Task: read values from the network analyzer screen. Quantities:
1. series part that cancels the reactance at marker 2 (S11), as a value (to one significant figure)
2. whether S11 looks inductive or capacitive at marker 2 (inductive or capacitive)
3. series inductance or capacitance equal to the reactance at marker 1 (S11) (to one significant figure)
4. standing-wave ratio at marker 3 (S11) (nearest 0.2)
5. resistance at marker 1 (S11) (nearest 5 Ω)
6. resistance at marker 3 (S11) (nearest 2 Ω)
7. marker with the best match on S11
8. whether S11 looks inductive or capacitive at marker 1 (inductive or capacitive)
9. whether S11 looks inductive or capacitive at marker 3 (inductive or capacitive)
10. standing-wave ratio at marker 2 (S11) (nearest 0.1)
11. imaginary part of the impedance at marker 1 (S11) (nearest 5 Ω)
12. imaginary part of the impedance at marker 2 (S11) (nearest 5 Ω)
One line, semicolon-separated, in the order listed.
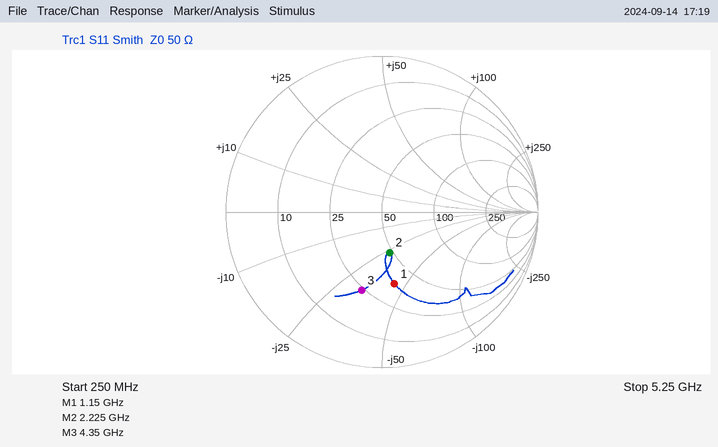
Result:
2 nH; capacitive; 3 pF; 3.2; 35 Ω; 24 Ω; marker 2; capacitive; capacitive; 1.7; -45 Ω; -25 Ω
